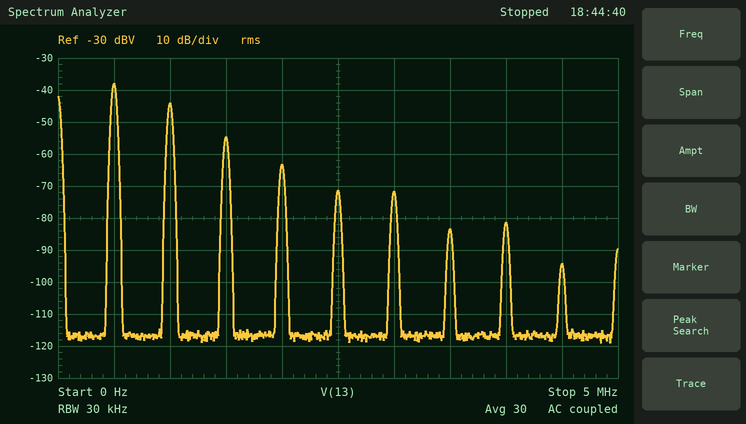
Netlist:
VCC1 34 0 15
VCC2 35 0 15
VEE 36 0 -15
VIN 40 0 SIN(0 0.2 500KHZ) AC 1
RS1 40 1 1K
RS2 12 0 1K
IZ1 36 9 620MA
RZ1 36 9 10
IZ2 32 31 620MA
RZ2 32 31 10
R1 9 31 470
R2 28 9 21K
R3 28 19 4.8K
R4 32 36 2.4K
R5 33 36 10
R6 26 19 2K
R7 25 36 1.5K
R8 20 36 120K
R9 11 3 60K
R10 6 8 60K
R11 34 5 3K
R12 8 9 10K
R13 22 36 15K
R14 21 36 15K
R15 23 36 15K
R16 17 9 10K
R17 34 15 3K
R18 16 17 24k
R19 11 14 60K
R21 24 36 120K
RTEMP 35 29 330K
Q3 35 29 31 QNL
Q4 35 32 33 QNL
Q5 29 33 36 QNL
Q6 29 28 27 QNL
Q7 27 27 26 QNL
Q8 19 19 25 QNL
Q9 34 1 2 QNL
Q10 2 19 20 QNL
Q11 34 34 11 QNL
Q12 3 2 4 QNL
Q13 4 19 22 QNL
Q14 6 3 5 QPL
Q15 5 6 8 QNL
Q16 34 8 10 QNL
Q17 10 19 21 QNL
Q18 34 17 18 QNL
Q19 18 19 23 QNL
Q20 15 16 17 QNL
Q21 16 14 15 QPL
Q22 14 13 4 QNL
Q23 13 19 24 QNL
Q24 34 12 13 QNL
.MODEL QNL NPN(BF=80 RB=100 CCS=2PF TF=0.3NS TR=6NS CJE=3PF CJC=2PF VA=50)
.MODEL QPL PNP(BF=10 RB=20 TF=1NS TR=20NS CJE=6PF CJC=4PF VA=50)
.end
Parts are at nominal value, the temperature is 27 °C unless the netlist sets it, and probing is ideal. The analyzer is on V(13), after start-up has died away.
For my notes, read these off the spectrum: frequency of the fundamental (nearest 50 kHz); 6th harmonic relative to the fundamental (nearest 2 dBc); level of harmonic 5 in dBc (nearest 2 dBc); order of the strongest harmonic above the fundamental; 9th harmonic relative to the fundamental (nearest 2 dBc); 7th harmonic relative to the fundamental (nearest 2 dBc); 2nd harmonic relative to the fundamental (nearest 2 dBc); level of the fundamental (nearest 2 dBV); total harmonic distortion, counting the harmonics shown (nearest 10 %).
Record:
500 kHz
-34 dBc
-34 dBc
2
-56 dBc
-46 dBc
-6 dBc
-38 dBV
50 %
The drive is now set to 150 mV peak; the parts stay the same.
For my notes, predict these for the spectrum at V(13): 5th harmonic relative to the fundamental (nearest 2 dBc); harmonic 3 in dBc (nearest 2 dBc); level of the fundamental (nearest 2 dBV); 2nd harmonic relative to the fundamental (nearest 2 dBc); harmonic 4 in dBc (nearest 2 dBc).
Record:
-36 dBc
-18 dBc
-40 dBV
-8 dBc
-28 dBc
